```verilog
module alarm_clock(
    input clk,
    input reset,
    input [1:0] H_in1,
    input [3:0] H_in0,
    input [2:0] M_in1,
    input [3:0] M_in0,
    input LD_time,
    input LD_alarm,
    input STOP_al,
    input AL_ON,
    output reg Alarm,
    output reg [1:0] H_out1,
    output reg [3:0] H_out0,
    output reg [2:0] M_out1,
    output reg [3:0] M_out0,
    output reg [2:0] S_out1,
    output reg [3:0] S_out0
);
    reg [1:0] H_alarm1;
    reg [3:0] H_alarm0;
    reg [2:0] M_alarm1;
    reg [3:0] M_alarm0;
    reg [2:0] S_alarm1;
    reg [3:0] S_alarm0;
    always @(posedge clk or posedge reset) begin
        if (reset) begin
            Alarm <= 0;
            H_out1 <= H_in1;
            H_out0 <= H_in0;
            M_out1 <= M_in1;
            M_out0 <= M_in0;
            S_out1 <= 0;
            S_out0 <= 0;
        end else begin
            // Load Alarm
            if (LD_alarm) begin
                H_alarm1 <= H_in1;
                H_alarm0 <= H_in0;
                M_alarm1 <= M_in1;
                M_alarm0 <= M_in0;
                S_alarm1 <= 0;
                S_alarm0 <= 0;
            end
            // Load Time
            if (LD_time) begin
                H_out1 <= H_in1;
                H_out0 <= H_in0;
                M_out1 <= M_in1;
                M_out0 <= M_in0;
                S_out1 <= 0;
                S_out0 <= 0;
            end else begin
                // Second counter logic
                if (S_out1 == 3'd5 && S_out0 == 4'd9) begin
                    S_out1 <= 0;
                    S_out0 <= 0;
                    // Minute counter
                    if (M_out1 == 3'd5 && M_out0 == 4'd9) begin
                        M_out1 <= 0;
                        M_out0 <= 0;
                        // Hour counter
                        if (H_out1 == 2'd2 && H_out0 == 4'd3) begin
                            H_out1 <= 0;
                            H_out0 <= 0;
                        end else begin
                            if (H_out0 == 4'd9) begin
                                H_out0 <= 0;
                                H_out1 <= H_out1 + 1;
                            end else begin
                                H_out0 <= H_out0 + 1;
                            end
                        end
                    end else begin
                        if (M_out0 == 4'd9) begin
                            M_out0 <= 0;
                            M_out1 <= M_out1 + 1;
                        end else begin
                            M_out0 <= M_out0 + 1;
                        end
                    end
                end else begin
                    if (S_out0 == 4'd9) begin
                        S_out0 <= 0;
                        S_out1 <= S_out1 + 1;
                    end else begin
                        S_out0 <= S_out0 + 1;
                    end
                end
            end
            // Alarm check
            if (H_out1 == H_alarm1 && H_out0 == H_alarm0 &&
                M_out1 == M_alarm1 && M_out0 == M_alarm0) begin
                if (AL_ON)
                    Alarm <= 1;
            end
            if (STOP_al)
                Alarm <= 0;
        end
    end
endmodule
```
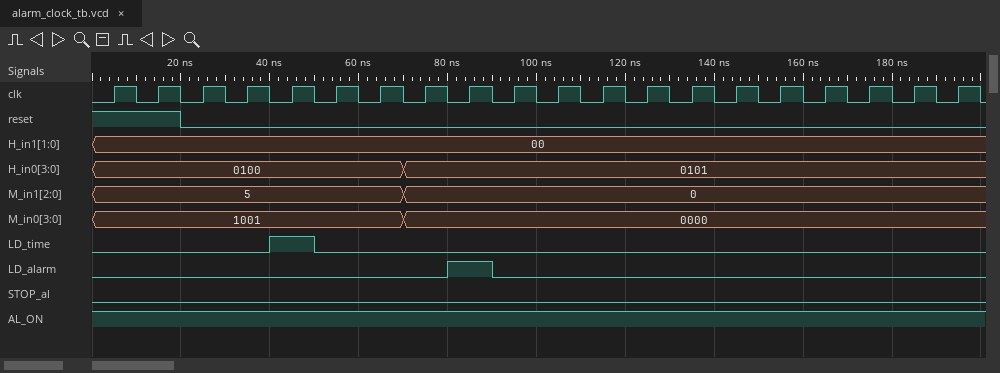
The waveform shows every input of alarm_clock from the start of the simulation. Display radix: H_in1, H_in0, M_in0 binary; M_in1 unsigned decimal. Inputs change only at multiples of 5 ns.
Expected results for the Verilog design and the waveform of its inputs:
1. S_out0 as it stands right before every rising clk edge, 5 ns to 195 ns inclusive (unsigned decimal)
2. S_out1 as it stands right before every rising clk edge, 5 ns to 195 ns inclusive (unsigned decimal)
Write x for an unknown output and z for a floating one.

0, 0, 0, 1, 2, 0, 1, 2, 3, 4, 5, 6, 7, 8, 9, 0, 1, 2, 3, 4
0, 0, 0, 0, 0, 0, 0, 0, 0, 0, 0, 0, 0, 0, 0, 1, 1, 1, 1, 1
